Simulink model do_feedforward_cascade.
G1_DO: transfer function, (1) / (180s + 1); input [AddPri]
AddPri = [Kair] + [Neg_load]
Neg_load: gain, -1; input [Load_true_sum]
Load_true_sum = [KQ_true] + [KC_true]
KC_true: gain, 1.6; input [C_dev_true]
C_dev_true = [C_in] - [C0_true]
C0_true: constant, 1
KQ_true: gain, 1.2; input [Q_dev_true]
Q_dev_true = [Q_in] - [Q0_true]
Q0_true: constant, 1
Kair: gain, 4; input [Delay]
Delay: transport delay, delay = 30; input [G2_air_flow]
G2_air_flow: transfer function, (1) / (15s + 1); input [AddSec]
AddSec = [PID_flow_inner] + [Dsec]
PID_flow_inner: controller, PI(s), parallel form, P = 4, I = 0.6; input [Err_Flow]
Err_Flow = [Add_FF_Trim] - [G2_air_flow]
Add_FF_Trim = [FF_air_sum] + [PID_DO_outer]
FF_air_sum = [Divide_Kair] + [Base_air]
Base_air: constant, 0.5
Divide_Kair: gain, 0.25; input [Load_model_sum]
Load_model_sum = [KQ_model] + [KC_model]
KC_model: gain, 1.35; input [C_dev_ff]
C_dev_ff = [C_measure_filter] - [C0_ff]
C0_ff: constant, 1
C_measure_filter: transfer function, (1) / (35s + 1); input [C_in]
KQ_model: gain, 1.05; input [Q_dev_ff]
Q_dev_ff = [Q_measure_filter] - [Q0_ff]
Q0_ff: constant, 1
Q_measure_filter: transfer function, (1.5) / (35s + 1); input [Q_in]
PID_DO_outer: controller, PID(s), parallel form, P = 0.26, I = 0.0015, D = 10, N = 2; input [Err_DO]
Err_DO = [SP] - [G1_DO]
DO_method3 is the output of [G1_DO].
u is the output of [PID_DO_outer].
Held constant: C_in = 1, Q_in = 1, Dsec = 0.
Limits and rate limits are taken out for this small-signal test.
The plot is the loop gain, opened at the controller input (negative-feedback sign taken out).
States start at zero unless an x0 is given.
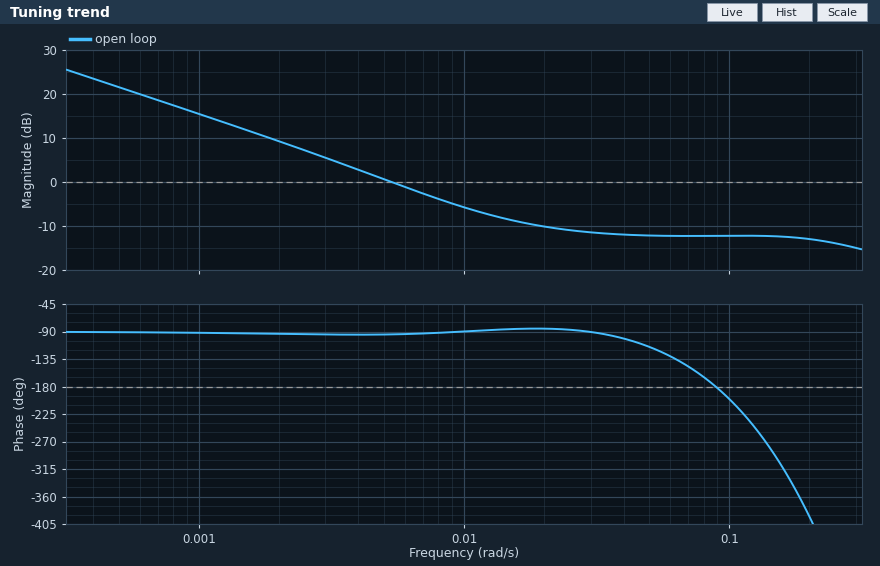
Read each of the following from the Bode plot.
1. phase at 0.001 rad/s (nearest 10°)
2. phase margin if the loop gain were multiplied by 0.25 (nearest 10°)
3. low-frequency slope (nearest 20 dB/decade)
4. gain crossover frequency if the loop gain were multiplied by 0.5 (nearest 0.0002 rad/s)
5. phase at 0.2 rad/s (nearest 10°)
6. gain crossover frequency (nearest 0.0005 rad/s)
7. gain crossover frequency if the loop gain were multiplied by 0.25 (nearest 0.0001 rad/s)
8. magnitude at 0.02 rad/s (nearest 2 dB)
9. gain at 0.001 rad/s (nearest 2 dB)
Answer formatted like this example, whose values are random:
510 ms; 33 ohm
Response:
-90°; 90°; -20 dB/decade; 0.0028 rad/s; -390°; 0.0055 rad/s; 0.0015 rad/s; -10 dB; 16 dB
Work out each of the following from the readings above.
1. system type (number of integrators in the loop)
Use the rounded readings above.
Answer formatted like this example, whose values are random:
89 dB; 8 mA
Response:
1
